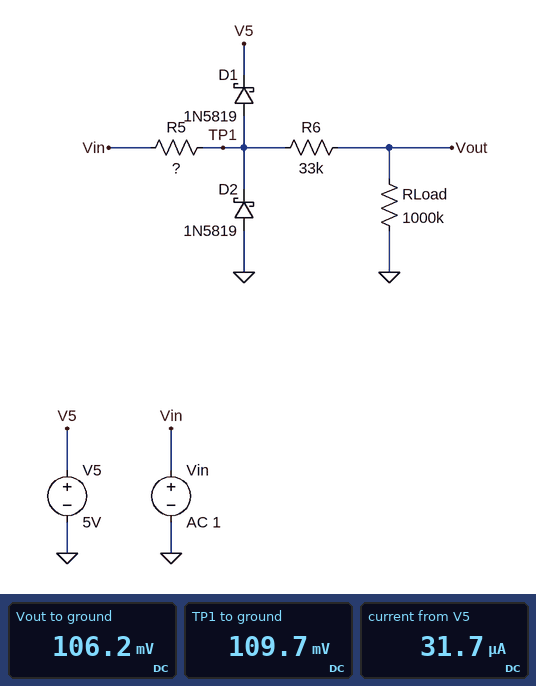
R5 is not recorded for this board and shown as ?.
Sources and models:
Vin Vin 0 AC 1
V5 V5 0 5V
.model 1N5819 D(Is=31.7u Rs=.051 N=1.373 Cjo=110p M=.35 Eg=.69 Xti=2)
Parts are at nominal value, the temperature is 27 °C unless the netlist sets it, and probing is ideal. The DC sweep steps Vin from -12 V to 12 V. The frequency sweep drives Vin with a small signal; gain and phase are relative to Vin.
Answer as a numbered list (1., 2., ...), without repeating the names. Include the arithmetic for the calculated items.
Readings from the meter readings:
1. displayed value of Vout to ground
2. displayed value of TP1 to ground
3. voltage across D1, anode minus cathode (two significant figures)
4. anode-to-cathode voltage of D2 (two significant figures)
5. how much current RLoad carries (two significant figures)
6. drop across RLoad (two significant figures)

1. 106.2 mV
2. 109.7 mV
3. 109.7 mV - 5 V = -4.9 V
4. 0 V - 109.7 mV = -110 mV
5. (106.2 mV) / 1 MΩ = 110 nA
6. 106.2 mV = 110 mV
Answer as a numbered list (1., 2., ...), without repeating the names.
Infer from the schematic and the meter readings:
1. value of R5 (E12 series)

1. 82 kΩ
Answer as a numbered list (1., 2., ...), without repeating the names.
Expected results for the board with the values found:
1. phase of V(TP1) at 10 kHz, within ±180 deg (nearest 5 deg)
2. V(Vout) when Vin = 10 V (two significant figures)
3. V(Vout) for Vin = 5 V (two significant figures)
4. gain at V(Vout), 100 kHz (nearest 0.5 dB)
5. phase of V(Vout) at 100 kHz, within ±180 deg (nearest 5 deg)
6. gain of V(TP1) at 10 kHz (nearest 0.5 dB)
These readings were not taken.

1. -10 deg
2. 4.9 V
3. 4.5 V
4. -20.0 dB
5. -65 deg
6. -13.0 dB
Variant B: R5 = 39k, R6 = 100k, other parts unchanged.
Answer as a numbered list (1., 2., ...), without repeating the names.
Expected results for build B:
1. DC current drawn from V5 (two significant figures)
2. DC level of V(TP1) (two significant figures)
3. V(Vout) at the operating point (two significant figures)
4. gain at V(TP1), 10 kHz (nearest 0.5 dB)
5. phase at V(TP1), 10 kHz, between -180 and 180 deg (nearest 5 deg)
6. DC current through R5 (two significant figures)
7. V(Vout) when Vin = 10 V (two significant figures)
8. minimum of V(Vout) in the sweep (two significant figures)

1. 32 µA
2. 91 mV
3. 83 mV
4. -11.5 dB
5. -5 deg
6. 2.3 µA
7. 4.6 V
8. -73 mV
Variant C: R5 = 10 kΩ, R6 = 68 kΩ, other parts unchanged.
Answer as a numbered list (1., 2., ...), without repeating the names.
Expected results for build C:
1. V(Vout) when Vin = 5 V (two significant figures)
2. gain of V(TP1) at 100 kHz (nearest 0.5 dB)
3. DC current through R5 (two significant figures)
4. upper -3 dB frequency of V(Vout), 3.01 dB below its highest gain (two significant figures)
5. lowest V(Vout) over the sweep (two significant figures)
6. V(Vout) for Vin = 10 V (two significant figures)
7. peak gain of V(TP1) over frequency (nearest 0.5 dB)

1. 4.6 V
2. -9.0 dB
3. 5.9 µA
4. 260 kHz
5. -120 mV
6. 4.8 V
7. -8.5 dB
